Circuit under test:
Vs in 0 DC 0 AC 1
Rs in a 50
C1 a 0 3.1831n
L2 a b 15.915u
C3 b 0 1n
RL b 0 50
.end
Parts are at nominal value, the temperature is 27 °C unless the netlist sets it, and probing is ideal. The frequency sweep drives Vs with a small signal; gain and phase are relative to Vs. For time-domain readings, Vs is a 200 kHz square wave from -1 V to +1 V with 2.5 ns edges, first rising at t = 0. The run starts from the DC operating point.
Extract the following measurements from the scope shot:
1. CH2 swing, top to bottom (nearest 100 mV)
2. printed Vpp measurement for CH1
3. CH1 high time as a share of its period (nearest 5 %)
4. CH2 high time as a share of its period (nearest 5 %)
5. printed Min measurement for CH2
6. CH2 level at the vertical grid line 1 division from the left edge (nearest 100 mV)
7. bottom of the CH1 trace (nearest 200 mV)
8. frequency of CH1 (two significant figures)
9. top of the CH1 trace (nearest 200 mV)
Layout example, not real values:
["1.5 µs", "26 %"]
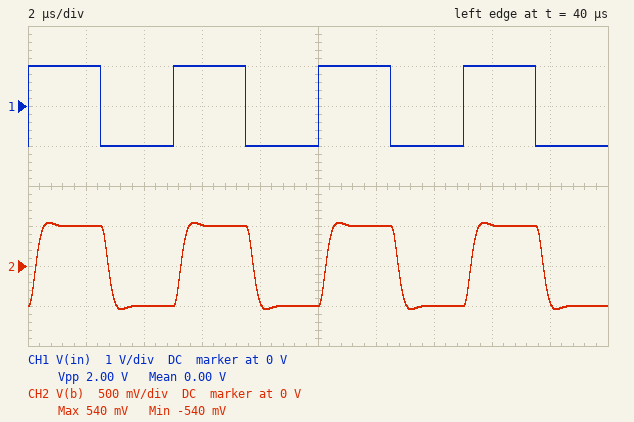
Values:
["1.1 V", "2.00 V", "50 %", "50 %", "-540 mV", "500 mV", "-1.0 V", "200 kHz", "1.0 V"]
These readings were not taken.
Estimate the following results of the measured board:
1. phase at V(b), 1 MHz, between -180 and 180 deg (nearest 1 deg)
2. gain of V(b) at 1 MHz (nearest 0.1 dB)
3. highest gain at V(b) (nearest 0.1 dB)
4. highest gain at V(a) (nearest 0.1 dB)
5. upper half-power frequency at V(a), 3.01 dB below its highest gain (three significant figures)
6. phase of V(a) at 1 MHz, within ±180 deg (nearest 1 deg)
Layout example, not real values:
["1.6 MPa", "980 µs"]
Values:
["-103 deg", "-8.8 dB", "-6.0 dB", "-2.6 dB", "1.88 MHz", "-24 deg"]
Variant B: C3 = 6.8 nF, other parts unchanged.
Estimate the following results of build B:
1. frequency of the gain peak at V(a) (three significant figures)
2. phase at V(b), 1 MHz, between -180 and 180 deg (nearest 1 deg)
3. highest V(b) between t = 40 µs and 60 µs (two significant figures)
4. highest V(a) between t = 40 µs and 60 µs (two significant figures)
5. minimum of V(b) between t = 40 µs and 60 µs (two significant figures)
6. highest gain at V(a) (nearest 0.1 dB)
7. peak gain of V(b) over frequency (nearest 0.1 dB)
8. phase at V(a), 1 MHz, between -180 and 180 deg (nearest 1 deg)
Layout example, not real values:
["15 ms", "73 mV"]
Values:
["926 kHz", "-169 deg", "580 mV", "800 mV", "-580 mV", "-1.0 dB", "-6.0 dB", "-20 deg"]
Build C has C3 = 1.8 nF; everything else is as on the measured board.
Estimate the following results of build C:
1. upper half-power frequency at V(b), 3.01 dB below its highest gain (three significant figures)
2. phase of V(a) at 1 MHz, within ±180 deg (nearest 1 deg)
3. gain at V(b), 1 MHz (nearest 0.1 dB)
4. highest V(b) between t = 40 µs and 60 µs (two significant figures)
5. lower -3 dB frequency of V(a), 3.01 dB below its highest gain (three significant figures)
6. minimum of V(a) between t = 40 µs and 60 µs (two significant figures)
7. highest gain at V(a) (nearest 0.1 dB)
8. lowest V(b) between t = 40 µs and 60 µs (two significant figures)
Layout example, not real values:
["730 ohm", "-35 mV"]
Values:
["1.05 MHz", "-21 deg", "-8.6 dB", "560 mV", "258 kHz", "-820 mV", "-2.5 dB", "-560 mV"]
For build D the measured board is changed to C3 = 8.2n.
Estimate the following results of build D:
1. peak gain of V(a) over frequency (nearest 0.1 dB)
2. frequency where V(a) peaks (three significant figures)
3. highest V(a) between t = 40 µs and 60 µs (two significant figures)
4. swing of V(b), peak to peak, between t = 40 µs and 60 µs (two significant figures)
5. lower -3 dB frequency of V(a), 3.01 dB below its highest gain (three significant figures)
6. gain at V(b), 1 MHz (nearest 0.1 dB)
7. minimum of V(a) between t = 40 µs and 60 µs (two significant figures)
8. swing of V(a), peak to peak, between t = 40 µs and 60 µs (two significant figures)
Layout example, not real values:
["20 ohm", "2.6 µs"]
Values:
["-0.8 dB", "895 kHz", "800 mV", "1.1 V", "604 kHz", "-14.3 dB", "-800 mV", "1.6 V"]
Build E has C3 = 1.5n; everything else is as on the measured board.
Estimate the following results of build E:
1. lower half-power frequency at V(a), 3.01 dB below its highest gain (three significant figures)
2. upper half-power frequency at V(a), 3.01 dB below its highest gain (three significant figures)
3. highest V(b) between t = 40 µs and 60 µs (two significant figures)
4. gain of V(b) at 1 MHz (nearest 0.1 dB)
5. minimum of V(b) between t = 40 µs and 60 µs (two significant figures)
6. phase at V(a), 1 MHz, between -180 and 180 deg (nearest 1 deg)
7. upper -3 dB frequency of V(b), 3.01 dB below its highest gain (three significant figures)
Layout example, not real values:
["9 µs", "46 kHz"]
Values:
["220 kHz", "1.89 MHz", "550 mV", "-8.6 dB", "-550 mV", "-22 deg", "1.05 MHz"]
